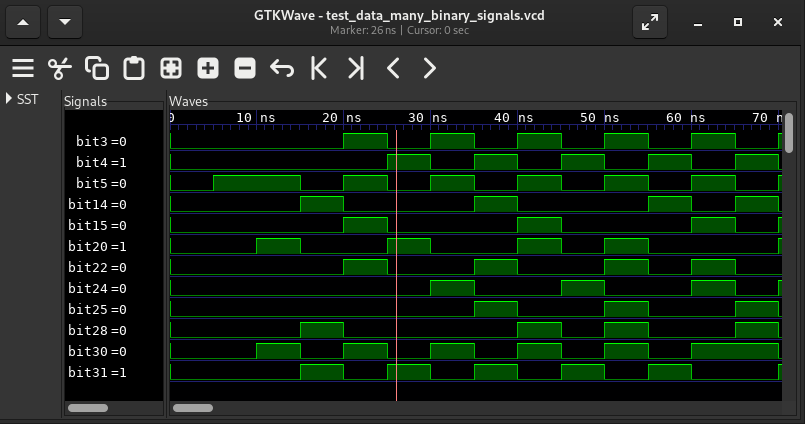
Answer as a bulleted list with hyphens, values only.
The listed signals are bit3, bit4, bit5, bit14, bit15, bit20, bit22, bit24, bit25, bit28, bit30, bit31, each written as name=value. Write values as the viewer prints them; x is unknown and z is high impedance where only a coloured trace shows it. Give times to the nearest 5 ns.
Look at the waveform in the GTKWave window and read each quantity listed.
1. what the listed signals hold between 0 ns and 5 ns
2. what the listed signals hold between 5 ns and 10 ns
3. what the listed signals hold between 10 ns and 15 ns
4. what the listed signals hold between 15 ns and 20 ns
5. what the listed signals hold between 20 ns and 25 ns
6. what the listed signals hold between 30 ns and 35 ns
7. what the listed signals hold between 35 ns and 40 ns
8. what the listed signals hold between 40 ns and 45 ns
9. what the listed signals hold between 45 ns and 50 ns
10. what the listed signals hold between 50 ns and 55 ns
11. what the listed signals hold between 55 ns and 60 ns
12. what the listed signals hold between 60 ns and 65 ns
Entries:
- bit3=0, bit4=0, bit5=0, bit14=0, bit15=0, bit20=0, bit22=0, bit24=0, bit25=0, bit28=0, bit30=0, bit31=0
- bit3=0, bit4=0, bit5=1, bit14=0, bit15=0, bit20=0, bit22=0, bit24=0, bit25=0, bit28=0, bit30=0, bit31=0
- bit3=0, bit4=0, bit5=1, bit14=0, bit15=0, bit20=1, bit22=0, bit24=0, bit25=0, bit28=0, bit30=1, bit31=0
- bit3=0, bit4=0, bit5=0, bit14=1, bit15=0, bit20=0, bit22=0, bit24=0, bit25=0, bit28=1, bit30=0, bit31=1
- bit3=1, bit4=0, bit5=1, bit14=0, bit15=1, bit20=0, bit22=1, bit24=0, bit25=0, bit28=0, bit30=1, bit31=0
- bit3=1, bit4=0, bit5=1, bit14=0, bit15=0, bit20=0, bit22=0, bit24=1, bit25=0, bit28=0, bit30=1, bit31=0
- bit3=0, bit4=1, bit5=0, bit14=1, bit15=0, bit20=0, bit22=1, bit24=0, bit25=1, bit28=0, bit30=0, bit31=1
- bit3=1, bit4=0, bit5=1, bit14=0, bit15=1, bit20=1, bit22=0, bit24=0, bit25=0, bit28=1, bit30=1, bit31=0
- bit3=0, bit4=1, bit5=0, bit14=0, bit15=0, bit20=0, bit22=0, bit24=1, bit25=0, bit28=0, bit30=0, bit31=1
- bit3=1, bit4=0, bit5=1, bit14=0, bit15=0, bit20=1, bit22=1, bit24=0, bit25=1, bit28=1, bit30=1, bit31=0
- bit3=0, bit4=1, bit5=0, bit14=1, bit15=0, bit20=0, bit22=0, bit24=0, bit25=0, bit28=0, bit30=0, bit31=1
- bit3=1, bit4=0, bit5=1, bit14=0, bit15=1, bit20=0, bit22=1, bit24=1, bit25=0, bit28=0, bit30=1, bit31=0
